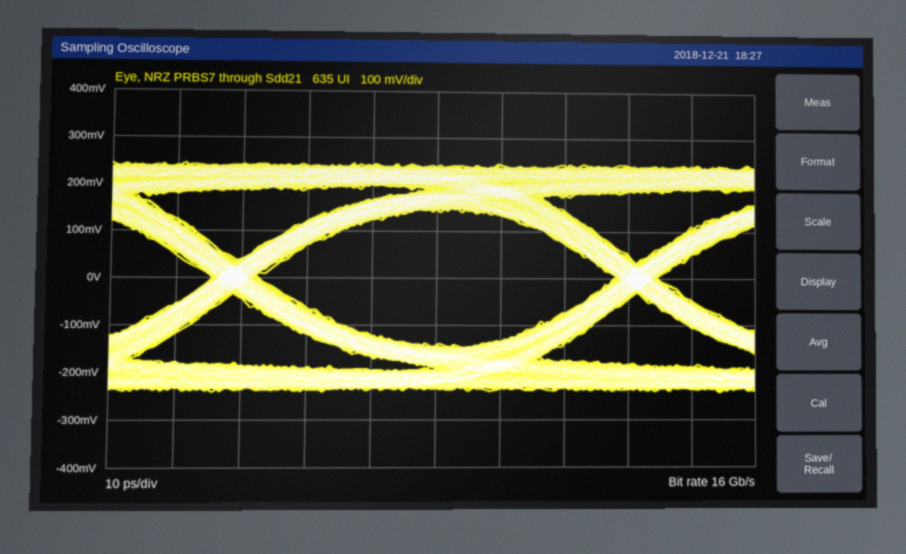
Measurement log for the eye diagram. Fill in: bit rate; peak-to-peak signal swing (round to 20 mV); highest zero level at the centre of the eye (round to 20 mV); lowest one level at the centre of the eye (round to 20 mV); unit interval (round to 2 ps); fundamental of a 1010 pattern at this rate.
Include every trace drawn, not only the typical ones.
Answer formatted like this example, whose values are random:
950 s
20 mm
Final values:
16 Gb/s
480 mV
-140 mV
140 mV
62 ps
8 GHz
